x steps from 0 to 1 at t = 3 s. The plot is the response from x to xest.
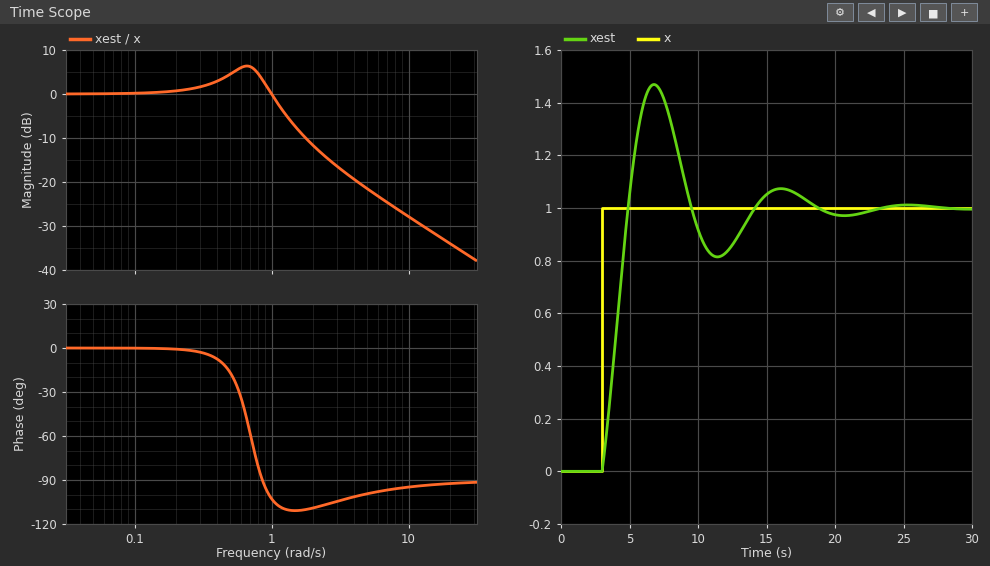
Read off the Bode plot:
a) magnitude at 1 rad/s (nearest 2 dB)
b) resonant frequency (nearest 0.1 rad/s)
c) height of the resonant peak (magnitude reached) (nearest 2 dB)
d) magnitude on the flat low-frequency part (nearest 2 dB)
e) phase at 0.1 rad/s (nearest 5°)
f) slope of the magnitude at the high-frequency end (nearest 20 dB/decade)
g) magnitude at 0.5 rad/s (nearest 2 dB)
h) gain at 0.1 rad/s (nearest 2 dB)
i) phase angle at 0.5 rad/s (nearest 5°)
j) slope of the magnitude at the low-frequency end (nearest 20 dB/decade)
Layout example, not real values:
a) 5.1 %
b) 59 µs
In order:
a) 0 dB
b) 0.7 rad/s
c) 6 dB
d) 0 dB
e) 0°
f) -20 dB/decade
g) 4 dB
h) 0 dB
i) -15°
j) 0 dB/decade
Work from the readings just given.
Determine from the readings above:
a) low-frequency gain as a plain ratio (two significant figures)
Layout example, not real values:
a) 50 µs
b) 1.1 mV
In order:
a) 1.0
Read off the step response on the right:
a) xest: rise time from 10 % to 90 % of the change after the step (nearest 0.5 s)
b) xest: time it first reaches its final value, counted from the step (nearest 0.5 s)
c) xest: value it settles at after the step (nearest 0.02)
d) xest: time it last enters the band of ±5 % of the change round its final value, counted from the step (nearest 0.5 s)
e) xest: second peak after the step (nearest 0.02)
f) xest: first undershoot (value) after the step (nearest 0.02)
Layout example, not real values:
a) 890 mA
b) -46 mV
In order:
a) 1.5 s
b) 2.0 s
c) 1.00
d) 14.5 s
e) 1.08
f) 0.82
